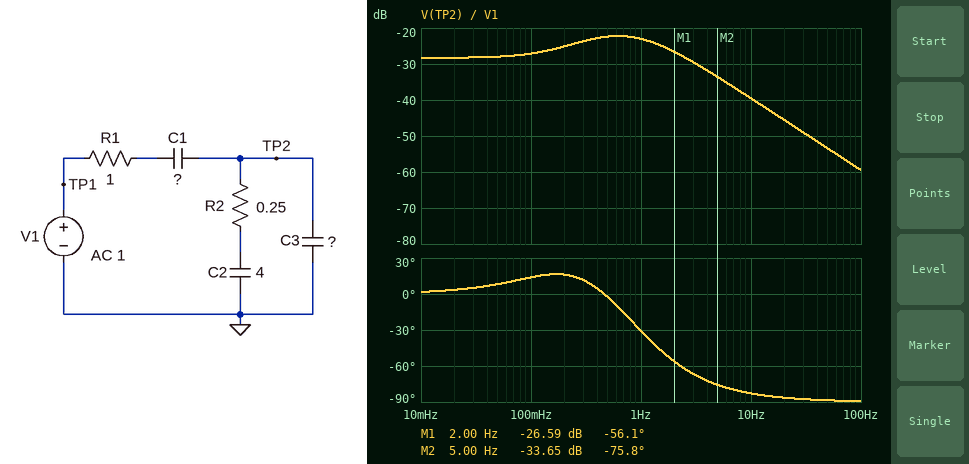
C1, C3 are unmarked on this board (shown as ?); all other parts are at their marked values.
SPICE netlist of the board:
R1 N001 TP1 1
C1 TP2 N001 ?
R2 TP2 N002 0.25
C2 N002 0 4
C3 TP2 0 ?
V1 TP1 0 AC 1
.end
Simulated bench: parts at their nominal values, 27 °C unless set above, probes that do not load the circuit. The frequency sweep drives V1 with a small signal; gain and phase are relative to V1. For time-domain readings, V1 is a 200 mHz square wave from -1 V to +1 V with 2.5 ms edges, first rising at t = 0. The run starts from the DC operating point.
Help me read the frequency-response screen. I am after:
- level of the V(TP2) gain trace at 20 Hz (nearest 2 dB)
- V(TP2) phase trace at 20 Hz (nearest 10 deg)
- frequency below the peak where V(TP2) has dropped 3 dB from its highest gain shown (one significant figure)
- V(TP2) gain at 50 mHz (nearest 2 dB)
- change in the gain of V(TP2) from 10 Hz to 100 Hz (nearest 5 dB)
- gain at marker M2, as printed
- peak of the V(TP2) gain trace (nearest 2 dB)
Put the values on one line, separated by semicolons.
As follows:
-46 dB; -90 deg; 200 mHz; -28 dB; -20 dB; -33.65 dB; -22 dB
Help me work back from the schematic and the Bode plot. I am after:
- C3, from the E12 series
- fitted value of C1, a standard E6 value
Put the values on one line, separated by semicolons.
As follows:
1.5 F; 220 mF
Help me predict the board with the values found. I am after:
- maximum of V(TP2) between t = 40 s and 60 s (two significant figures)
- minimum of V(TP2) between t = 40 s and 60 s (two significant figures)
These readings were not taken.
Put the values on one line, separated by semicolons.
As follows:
140 mV; -59 mV
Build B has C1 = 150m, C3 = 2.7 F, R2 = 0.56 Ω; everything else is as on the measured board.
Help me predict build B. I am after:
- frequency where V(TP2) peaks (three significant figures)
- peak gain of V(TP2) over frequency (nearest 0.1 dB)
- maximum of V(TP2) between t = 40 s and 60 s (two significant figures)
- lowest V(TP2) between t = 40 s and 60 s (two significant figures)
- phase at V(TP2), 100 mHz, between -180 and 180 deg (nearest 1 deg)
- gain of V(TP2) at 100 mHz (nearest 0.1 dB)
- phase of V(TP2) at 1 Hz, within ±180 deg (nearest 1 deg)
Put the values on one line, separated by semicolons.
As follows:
410 mHz; -26.7 dB; 81 mV; -37 mV; 19 deg; -29.8 dB; -36 deg
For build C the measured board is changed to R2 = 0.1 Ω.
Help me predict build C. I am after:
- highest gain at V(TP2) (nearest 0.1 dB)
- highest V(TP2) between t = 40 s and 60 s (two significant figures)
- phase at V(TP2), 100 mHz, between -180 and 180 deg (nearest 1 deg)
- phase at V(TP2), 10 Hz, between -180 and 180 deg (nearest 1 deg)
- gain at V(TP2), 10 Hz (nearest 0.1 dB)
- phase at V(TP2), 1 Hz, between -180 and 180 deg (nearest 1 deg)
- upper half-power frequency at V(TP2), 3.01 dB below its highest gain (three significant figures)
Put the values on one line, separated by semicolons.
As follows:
-26.0 dB; 96 mV; 2 deg; -79 deg; -39.6 dB; -19 deg; 2.43 Hz
